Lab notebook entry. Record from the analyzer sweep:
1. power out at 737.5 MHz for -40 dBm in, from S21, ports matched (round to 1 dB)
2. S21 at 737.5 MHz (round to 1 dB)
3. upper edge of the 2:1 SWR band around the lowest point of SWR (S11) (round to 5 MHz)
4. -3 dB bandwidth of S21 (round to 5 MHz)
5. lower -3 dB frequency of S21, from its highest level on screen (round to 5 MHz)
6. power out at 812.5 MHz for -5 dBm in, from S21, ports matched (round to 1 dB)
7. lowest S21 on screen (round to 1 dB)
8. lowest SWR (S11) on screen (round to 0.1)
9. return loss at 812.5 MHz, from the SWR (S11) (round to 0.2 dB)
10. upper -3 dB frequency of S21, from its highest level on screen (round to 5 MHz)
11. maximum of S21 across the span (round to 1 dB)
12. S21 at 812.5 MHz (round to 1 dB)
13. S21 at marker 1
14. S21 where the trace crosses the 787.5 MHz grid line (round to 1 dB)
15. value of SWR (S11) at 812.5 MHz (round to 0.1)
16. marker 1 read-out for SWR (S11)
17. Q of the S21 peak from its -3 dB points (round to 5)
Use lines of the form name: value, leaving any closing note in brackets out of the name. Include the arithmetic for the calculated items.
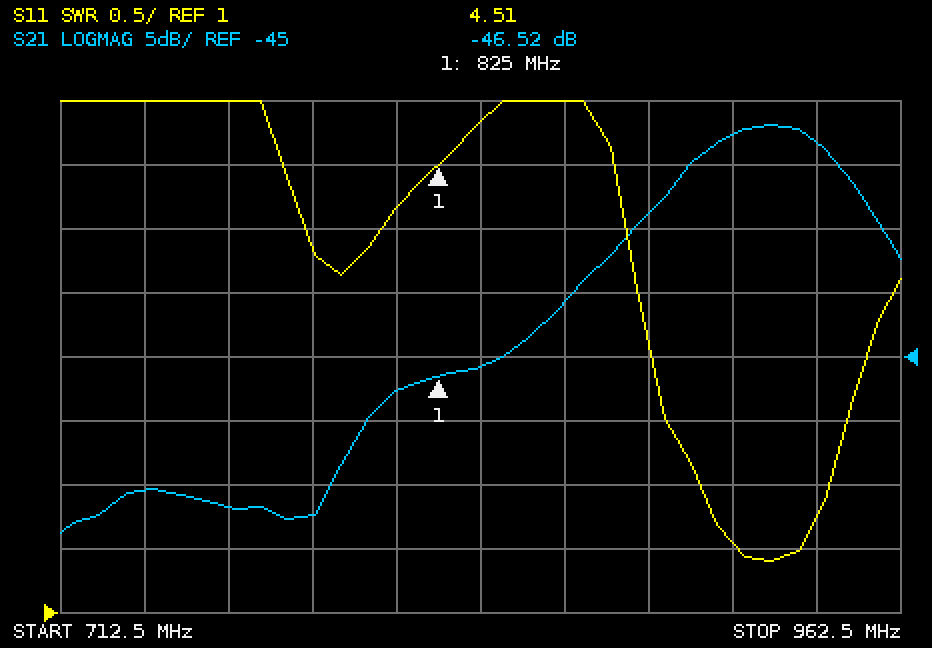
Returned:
power out at 737.5 MHz for -40 dBm in, from S21, ports matched: -40 dBm + (-55 dB) = -95 dBm
S21 at 737.5 MHz: -55 dB
upper edge of the 2:1 SWR band around the lowest point of SWR (S11): 940 MHz
-3 dB bandwidth of S21: 945 MHz − 900 MHz = 45 MHz
lower -3 dB frequency of S21, from its highest level on screen: 900 MHz
power out at 812.5 MHz for -5 dBm in, from S21, ports matched: -5 dBm + (-48 dB) = -53 dBm
lowest S21 on screen: -59 dB
lowest SWR (S11) on screen: 1.4
return loss at 812.5 MHz, from the SWR (S11): −20 log10((4.2 − 1)/(4.2 + 1)) ≈ 4.2 dB
upper -3 dB frequency of S21, from its highest level on screen: 945 MHz
maximum of S21 across the span: -27 dB
S21 at 812.5 MHz: -48 dB
S21 at marker 1: -46.52 dB
S21 where the trace crosses the 787.5 MHz grid line: -57 dB
value of SWR (S11) at 812.5 MHz: 4.2
marker 1 read-out for SWR: 4.51
Q of the S21 peak from its -3 dB points: 922.5 MHz / 45 MHz ≈ 20
